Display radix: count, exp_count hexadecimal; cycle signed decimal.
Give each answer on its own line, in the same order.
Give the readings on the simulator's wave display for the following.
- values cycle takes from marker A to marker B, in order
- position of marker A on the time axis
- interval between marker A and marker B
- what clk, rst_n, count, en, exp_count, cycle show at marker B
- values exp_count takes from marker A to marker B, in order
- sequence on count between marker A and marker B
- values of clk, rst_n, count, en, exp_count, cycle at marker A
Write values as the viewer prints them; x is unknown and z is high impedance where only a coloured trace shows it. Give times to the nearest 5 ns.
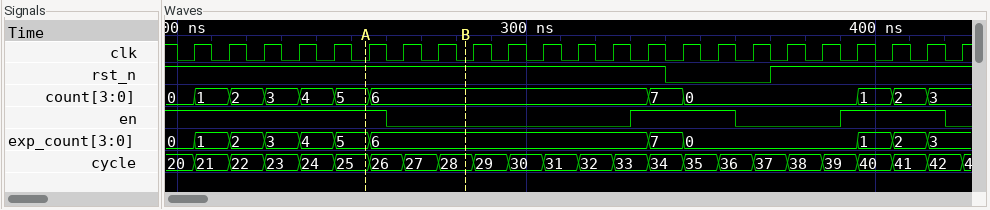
25, 26, 27, 28
255 ns
30 ns
clk=0, rst_n=1, count=6, en=0, exp_count=6, cycle=28
5, 6
5, 6
clk=0, rst_n=1, count=5, en=1, exp_count=5, cycle=25
